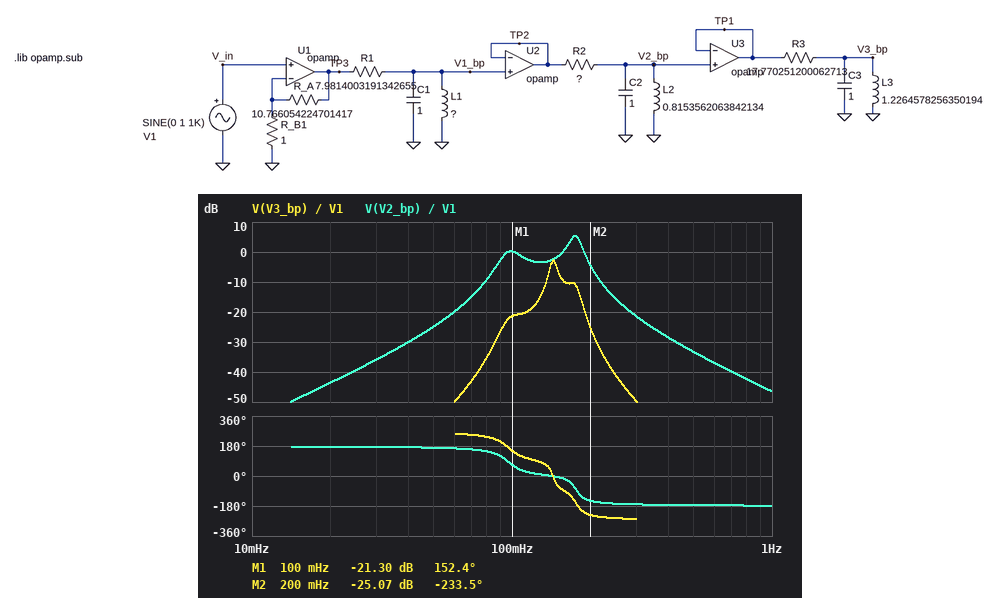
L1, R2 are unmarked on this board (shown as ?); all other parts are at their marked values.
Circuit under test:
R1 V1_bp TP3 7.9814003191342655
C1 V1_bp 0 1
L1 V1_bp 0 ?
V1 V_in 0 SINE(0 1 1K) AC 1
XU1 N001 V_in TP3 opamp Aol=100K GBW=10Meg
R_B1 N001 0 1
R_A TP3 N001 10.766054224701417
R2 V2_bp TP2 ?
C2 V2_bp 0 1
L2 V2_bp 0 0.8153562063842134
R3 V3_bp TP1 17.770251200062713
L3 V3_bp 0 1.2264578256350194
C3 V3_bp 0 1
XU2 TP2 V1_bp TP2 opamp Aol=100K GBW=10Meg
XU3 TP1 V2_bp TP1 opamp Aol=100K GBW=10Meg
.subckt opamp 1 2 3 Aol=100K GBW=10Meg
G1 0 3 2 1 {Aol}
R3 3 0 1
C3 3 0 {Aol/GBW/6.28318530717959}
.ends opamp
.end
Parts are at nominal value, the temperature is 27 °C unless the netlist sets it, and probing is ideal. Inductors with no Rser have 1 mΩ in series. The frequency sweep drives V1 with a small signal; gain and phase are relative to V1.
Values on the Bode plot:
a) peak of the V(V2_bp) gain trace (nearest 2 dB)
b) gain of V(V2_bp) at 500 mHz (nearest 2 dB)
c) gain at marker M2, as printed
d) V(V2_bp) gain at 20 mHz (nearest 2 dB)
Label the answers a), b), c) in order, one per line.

a) 6 dB
b) -34 dB
c) -25.07 dB
d) -44 dB
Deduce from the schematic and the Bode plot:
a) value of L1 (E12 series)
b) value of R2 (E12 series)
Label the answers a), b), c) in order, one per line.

a) 2.7 H
b) 8.2 Ω
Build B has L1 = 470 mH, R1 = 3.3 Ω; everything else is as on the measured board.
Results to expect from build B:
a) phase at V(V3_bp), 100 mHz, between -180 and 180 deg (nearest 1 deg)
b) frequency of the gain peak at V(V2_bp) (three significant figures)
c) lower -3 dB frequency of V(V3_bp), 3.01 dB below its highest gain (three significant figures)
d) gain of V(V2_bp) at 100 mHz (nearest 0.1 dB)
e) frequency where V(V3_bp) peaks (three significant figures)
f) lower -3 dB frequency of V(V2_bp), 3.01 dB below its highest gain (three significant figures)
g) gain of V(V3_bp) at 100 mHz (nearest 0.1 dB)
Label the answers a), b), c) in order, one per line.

a) -107 deg
b) 178 mHz
c) 141 mHz
d) -18.6 dB
e) 145 mHz
f) 169 mHz
g) -40.1 dB
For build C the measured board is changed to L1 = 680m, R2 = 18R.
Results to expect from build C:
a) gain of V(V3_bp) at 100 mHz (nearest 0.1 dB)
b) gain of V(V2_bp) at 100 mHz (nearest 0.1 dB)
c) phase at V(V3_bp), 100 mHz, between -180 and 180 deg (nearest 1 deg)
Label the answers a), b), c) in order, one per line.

a) -50.4 dB
b) -28.9 dB
c) -102 deg
